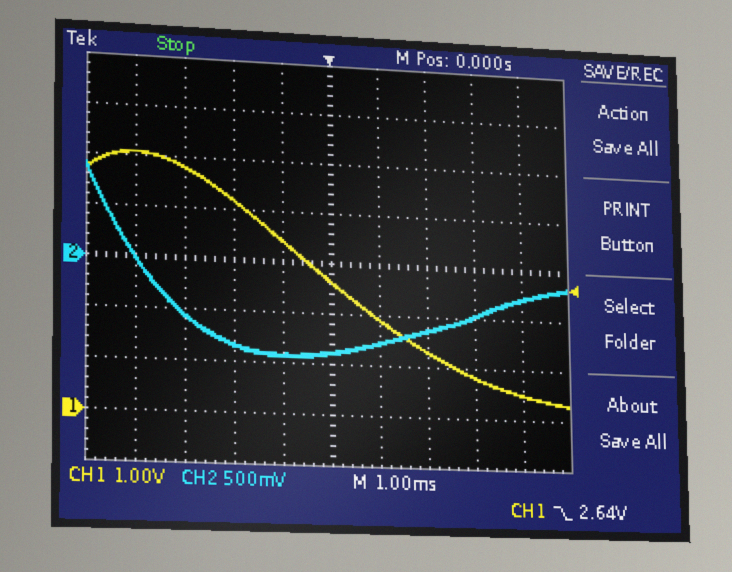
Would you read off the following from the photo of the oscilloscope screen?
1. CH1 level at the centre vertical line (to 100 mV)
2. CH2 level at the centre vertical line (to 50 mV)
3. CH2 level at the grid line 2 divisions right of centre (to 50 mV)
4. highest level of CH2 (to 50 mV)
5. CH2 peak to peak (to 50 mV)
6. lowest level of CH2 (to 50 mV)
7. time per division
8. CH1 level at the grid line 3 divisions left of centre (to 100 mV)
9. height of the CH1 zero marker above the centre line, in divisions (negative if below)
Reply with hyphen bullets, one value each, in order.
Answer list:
- 2.6 V
- -900 mV
- -650 mV
- 900 mV
- 1.85 V
- -950 mV
- 1 ms
- 4.8 V
- -3.0 div
